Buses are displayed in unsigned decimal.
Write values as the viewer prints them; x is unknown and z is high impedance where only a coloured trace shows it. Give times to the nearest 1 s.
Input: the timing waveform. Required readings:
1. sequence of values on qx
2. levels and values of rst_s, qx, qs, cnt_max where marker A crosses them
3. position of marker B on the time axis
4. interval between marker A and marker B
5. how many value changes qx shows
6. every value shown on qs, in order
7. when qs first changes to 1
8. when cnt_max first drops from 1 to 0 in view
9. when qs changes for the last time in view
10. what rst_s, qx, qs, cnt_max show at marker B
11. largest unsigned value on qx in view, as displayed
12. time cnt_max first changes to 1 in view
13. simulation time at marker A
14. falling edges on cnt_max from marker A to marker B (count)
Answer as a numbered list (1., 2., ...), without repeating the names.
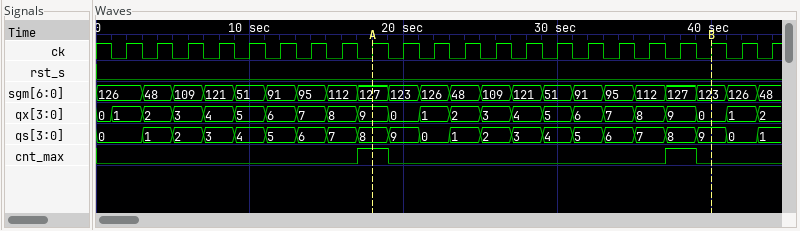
1. 0, 1, 2, 3, 4, 5, 6, 7, 8, 9, 0, 1, 2, 3, 4, 5, 6, 7, 8, 9, 0, 1, 2
2. rst_s=0, qx=9, qs=8, cnt_max=1
3. 40 s
4. 22 s
5. 22
6. 0, 1, 2, 3, 4, 5, 6, 7, 8, 9, 0, 1, 2, 3, 4, 5, 6, 7, 8, 9, 0, 1
7. 3 s
8. 19 s
9. 43 s
10. rst_s=0, qx=0, qs=9, cnt_max=0
11. 9
12. 17 s
13. 18 s
14. 2
